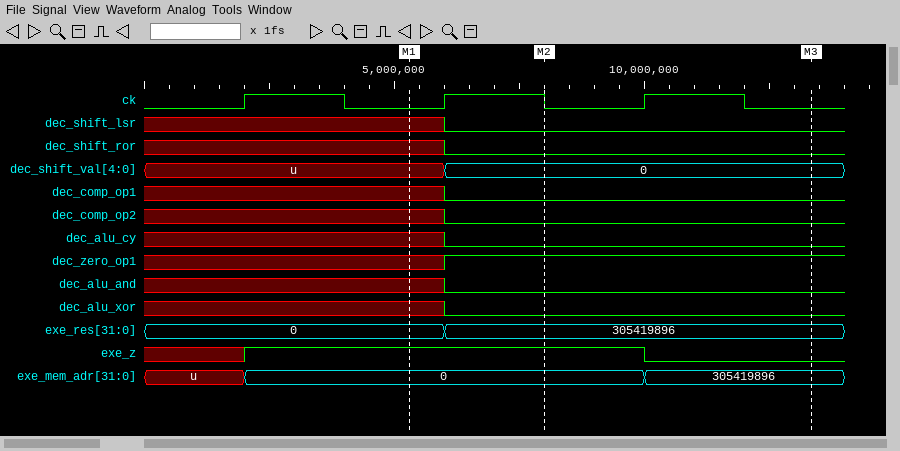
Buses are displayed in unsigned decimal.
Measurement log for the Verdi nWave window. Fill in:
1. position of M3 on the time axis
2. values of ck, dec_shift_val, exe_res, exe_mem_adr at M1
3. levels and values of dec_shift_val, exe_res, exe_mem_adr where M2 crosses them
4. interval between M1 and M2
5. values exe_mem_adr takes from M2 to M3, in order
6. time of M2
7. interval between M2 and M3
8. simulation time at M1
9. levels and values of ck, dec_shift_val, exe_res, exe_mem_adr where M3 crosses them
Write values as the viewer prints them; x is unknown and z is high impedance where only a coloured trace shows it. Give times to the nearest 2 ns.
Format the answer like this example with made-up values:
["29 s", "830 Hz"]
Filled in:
["14 ns", "ck=0, dec_shift_val=u, exe_res=0, exe_mem_adr=0", "dec_shift_val=0, exe_res=305419896, exe_mem_adr=0", "2 ns", "0, 305419896", "8 ns", "6 ns", "6 ns", "ck=0, dec_shift_val=0, exe_res=305419896, exe_mem_adr=305419896"]
